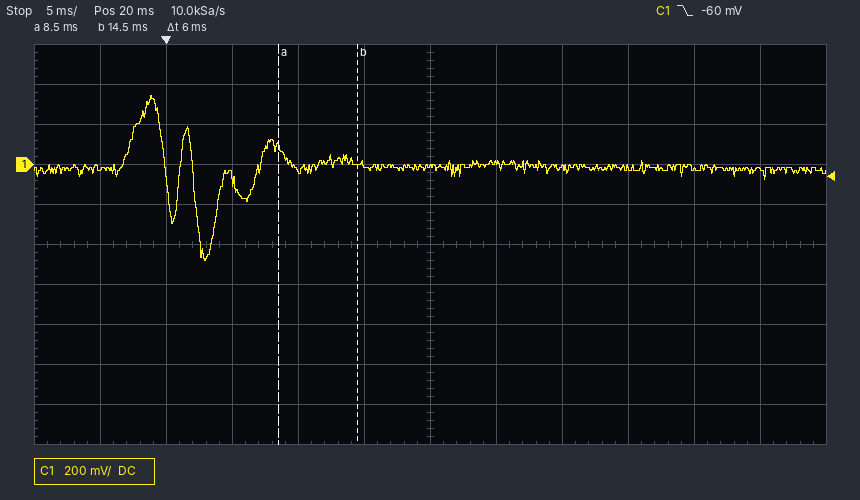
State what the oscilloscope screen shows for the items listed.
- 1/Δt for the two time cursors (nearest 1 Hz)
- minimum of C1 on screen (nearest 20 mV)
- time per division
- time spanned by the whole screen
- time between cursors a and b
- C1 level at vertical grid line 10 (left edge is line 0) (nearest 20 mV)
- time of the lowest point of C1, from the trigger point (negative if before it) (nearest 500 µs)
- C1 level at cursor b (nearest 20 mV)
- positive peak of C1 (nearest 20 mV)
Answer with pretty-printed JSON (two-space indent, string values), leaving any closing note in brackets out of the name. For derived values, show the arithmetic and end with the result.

{
  "1/Δt for the two time cursors": "1 / 6 ms ≈ 167 Hz",
  "minimum of C1 on screen": "-480 mV",
  "time per division": "5 ms",
  "time spanned by the whole screen": "60 ms",
  "time between cursors a and b": "6 ms",
  "C1 level at vertical grid line 10 (left edge is line 0)": "-20 mV",
  "time of the lowest point of C1, from the trigger point (negative if before it)": "+3.0 ms",
  "C1 level at cursor b": "0 mV",
  "positive peak of C1": "340 mV"
}
